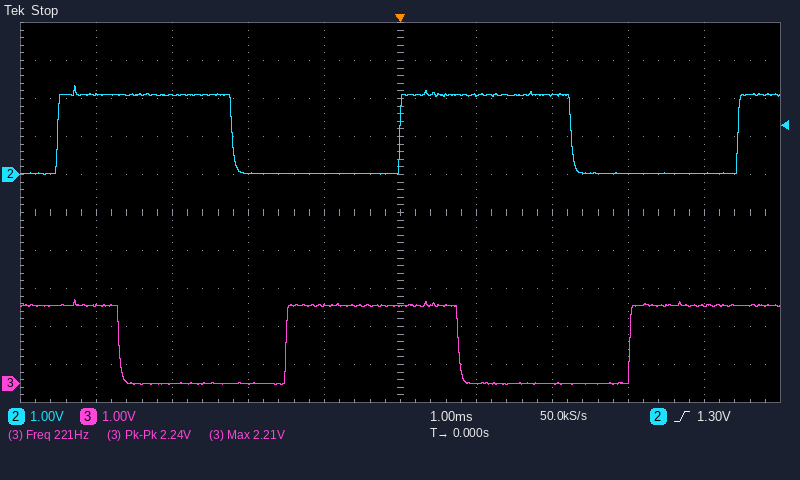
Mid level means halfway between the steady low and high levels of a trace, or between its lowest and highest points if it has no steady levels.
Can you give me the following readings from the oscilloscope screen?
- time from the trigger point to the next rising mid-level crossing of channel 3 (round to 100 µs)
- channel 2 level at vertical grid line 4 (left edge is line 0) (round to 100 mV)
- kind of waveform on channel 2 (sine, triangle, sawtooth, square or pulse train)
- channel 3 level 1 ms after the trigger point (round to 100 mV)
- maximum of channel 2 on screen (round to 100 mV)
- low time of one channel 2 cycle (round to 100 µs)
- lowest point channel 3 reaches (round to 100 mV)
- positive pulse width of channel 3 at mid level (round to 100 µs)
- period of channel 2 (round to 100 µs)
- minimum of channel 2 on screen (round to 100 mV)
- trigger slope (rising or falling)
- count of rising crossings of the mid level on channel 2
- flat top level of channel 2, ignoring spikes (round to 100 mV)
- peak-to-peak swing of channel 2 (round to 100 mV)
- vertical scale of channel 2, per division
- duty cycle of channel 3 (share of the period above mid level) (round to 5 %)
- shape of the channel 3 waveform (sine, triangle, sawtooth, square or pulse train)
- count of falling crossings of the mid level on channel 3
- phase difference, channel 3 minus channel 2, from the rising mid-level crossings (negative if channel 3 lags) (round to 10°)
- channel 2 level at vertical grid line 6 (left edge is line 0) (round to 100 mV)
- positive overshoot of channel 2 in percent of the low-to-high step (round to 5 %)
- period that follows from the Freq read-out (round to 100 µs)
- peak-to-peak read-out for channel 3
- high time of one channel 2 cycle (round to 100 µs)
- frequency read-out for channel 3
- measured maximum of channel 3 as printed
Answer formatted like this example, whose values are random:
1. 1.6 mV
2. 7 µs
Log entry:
1. 3.0 ms
2. 0.0 V
3. square
4. 0.0 V
5. 2.3 V
6. 2.2 ms
7. 0.0 V
8. 2.3 ms
9. 4.5 ms
10. 0.0 V
11. rising
12. 3
13. 2.1 V
14. 2.3 V
15. 1 V
16. 50 %
17. square
18. 2
19. +120°
20. 2.1 V
21. 10 %
22. 4.5 ms
23. 2.24 V
24. 2.3 ms
25. 221 Hz
26. 2.21 V
